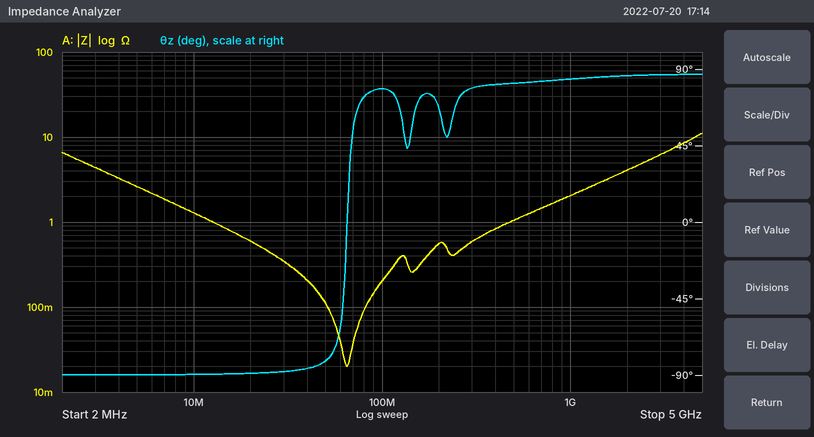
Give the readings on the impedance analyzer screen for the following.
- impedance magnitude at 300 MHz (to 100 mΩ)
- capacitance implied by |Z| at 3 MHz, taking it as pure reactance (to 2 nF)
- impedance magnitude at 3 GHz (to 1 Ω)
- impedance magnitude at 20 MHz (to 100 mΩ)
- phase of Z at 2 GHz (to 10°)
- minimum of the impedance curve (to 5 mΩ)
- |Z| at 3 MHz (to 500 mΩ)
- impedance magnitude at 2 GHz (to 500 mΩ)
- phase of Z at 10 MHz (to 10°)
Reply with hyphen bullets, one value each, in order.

- 600 mΩ
- 12 nF
- 6 Ω
- 600 mΩ
- 90°
- 20 mΩ
- 4.5 Ω
- 4.0 Ω
- -90°
